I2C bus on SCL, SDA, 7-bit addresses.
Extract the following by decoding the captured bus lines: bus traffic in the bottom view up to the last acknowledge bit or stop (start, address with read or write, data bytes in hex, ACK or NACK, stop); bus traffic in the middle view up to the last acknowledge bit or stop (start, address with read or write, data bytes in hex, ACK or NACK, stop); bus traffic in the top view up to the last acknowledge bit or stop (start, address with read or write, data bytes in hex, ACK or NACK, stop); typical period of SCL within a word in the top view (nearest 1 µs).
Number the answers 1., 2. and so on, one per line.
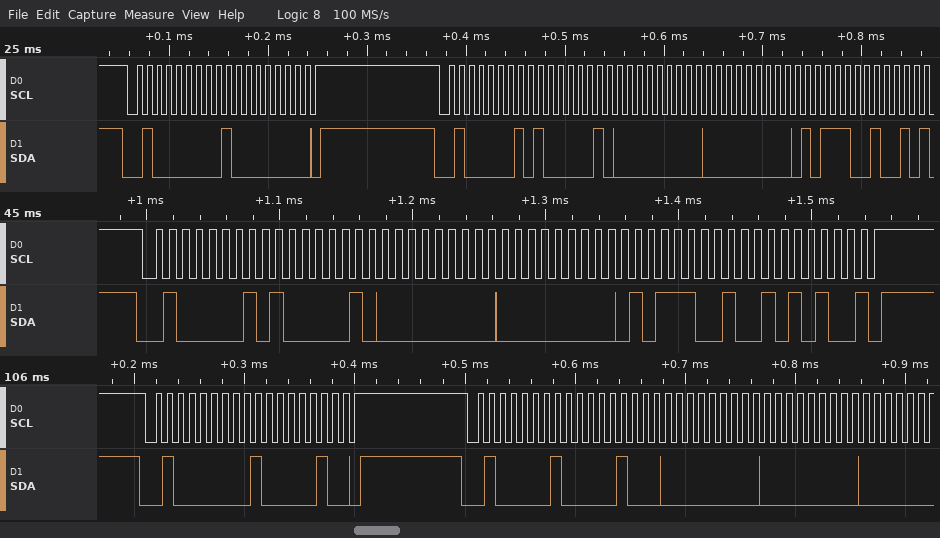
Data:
1. start, address 20 write ACK, 82 ACK, stop, start, address 20 read ACK, 08 ACK, 00 ACK, 00 ACK
2. start, address 20 read ACK, 82 ACK, 00 ACK, 00 ACK, B9 ACK, 54 NACK, stop
3. start, address 20 write ACK, 80 ACK, stop, start, address 20 read ACK, 82 ACK, 00 ACK, 00 ACK, B9 ACK
4. 10 µs
